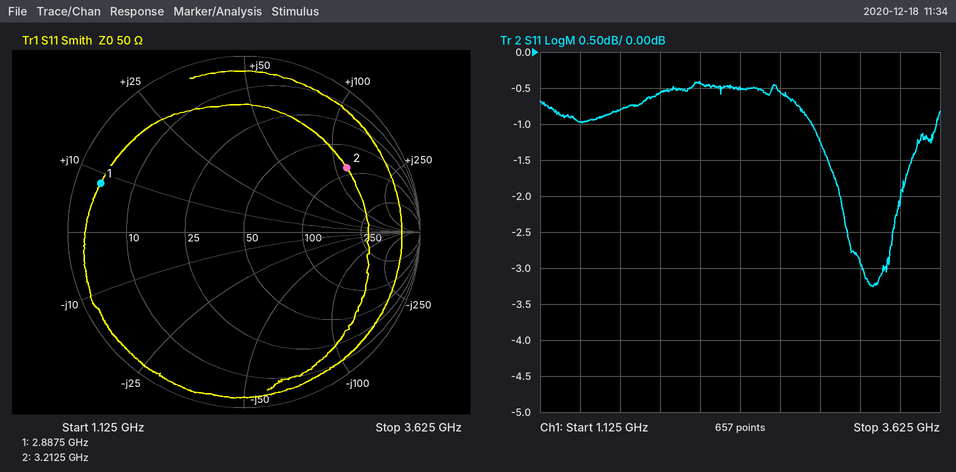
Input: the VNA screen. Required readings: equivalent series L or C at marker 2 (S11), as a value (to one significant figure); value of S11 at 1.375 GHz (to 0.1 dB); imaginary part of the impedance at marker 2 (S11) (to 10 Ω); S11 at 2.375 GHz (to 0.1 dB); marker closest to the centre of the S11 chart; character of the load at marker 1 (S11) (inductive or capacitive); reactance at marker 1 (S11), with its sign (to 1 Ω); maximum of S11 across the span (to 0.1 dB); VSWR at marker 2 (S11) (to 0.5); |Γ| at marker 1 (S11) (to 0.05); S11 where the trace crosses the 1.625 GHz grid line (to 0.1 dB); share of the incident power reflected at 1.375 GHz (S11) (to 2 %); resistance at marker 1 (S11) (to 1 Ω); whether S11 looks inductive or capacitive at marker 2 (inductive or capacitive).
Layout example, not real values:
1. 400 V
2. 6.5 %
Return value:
1. 6 nH
2. -1.0 dB
3. +120 Ω
4. -0.5 dB
5. marker 2
6. inductive
7. +8 Ω
8. -0.4 dB
9. 5.5
10. 0.85
11. -0.8 dB
12. 80 %
13. 4 Ω
14. inductive
